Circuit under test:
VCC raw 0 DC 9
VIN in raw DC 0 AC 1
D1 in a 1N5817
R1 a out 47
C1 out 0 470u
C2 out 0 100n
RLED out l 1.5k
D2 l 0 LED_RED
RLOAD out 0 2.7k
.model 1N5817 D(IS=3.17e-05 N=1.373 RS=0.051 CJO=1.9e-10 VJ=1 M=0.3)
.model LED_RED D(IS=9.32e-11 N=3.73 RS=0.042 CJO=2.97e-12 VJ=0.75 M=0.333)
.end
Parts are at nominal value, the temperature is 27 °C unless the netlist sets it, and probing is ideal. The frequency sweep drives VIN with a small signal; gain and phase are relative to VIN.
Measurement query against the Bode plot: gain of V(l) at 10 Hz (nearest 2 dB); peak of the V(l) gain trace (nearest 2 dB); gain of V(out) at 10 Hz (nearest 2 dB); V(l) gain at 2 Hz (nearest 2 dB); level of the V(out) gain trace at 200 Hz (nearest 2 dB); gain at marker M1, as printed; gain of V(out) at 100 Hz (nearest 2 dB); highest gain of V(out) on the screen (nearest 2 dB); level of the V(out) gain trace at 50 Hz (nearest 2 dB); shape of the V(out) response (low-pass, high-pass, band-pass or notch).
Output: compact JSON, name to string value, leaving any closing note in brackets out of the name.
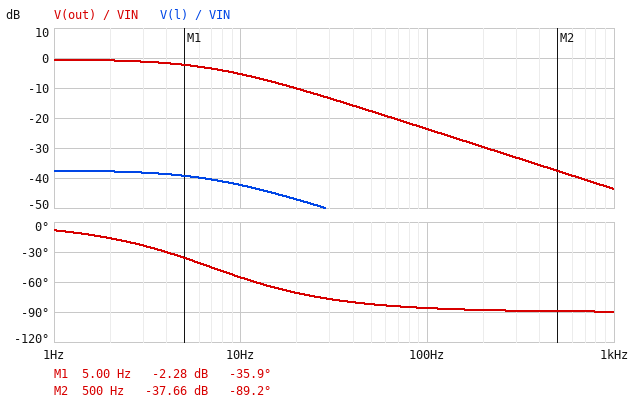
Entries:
{"gain of V(l) at 10 Hz": "-42 dB", "peak of the V(l) gain trace": "-38 dB", "gain of V(out) at 10 Hz": "-6 dB", "V(l) gain at 2 Hz": "-38 dB", "level of the V(out) gain trace at 200 Hz": "-30 dB", "gain at marker M1, as printed": "-2.28 dB", "gain of V(out) at 100 Hz": "-24 dB", "highest gain of V(out) on the screen": "0 dB", "level of the V(out) gain trace at 50 Hz": "-18 dB", "shape of the V(out) response": "low-pass"}
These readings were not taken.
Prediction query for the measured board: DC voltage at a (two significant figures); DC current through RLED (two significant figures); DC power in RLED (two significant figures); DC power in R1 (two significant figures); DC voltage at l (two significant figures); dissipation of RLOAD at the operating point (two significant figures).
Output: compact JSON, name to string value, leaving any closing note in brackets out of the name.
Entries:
{"DC voltage at a": "8.8 V", "DC current through RLED": "4.5 mA", "DC power in RLED": "30 mW", "DC power in R1": "2.7 mW", "DC voltage at l": "1.7 V", "dissipation of RLOAD at the operating point": "26 mW"}
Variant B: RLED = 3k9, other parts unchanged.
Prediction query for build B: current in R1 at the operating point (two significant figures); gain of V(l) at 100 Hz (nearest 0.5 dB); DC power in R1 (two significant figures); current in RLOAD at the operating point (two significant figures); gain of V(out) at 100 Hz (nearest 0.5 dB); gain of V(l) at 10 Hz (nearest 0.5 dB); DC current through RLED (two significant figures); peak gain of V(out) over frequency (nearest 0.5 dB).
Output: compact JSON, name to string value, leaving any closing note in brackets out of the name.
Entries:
{"current in R1 at the operating point": "5.0 mA", "gain of V(l) at 100 Hz": "-61.5 dB", "DC power in R1": "1.2 mW", "current in RLOAD at the operating point": "3.2 mA", "gain of V(out) at 100 Hz": "-24.0 dB", "gain of V(l) at 10 Hz": "-43.0 dB", "DC current through RLED": "1.8 mA", "peak gain of V(out) over frequency": "-0.5 dB"}
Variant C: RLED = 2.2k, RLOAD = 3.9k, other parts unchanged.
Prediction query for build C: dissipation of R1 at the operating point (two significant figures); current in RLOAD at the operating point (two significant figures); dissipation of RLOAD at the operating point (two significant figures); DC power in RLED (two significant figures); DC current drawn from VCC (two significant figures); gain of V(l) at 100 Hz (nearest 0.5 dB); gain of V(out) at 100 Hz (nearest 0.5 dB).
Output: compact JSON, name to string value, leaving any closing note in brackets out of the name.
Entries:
{"dissipation of R1 at the operating point": "1.3 mW", "current in RLOAD at the operating point": "2.2 mA", "dissipation of RLOAD at the operating point": "19 mW", "DC power in RLED": "22 mW", "DC current drawn from VCC": "5.3 mA", "gain of V(l) at 100 Hz": "-61.0 dB", "gain of V(out) at 100 Hz": "-24.0 dB"}
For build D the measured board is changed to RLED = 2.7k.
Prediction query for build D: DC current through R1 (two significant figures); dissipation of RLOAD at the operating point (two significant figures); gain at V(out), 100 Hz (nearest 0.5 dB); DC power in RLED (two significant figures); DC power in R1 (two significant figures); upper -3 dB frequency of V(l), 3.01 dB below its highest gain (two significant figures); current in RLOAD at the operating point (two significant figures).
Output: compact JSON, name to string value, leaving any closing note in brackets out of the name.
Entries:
{"DC current through R1": "5.7 mA", "dissipation of RLOAD at the operating point": "27 mW", "gain at V(out), 100 Hz": "-24.0 dB", "DC power in RLED": "18 mW", "DC power in R1": "1.5 mW", "upper -3 dB frequency of V(l), 3.01 dB below its highest gain": "6.6 Hz", "current in RLOAD at the operating point": "3.2 mA"}
